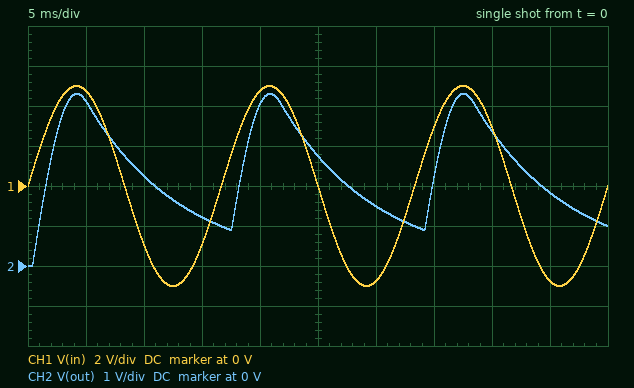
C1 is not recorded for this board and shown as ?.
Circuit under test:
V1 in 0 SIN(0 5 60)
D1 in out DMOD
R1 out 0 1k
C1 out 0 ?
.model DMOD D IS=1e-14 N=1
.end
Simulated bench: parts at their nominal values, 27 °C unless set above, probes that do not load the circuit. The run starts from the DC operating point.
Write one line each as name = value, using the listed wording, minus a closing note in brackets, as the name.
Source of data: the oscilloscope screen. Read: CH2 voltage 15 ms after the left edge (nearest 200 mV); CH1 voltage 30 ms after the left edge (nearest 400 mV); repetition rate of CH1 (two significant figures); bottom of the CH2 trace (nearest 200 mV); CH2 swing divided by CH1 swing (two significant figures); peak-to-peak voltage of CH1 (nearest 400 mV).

CH2 voltage 15 ms after the left edge = 1.2 V
CH1 voltage 30 ms after the left edge = -4.8 V
repetition rate of CH1 = 60 Hz
bottom of the CH2 trace = 0 V
CH2 swing divided by CH1 swing = 0.43
peak-to-peak voltage of CH1 = 10.0 V
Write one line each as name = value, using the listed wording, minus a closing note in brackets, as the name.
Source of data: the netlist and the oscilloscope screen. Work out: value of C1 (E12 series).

value of C1 = 8.2 µF
